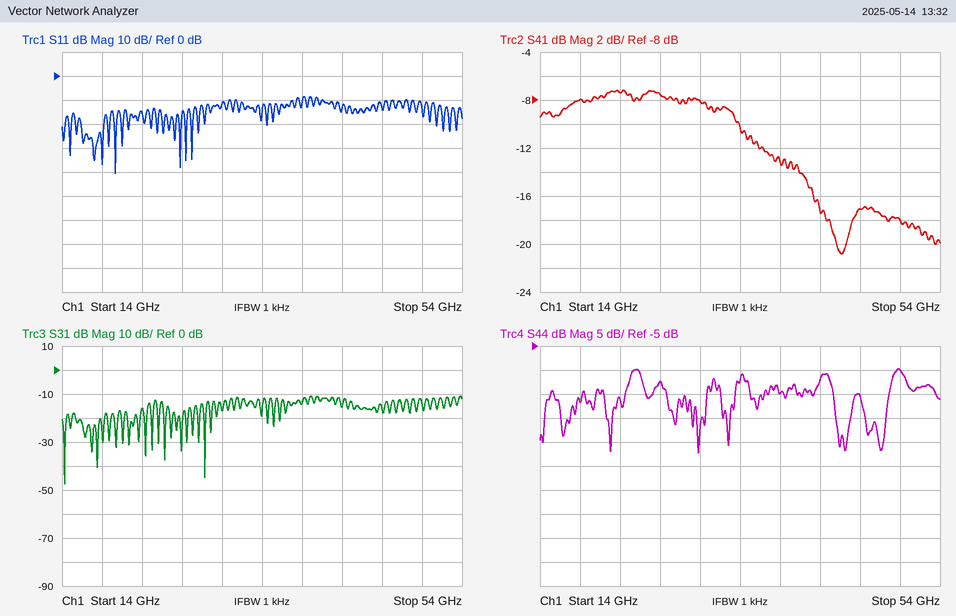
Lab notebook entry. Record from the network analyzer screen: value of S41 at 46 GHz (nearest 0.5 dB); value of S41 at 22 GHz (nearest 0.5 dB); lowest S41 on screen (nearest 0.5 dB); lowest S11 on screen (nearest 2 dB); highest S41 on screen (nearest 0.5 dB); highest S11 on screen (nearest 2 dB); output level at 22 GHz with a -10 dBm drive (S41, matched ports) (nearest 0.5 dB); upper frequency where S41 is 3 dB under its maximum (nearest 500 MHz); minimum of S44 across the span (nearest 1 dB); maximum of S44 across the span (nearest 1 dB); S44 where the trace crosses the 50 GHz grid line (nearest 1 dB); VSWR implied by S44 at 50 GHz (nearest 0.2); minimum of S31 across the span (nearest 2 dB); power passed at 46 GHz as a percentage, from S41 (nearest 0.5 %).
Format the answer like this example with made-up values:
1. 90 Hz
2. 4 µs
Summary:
1. -17.0 dB
2. -7.5 dB
3. -21.0 dB
4. -40 dB
5. -7.0 dB
6. -8 dB
7. -17.5 dBm
8. 34.0 GHz
9. -27 dB
10. -10 dB
11. -10 dB
12. 2.0
13. -48 dB
14. 2.0 %
